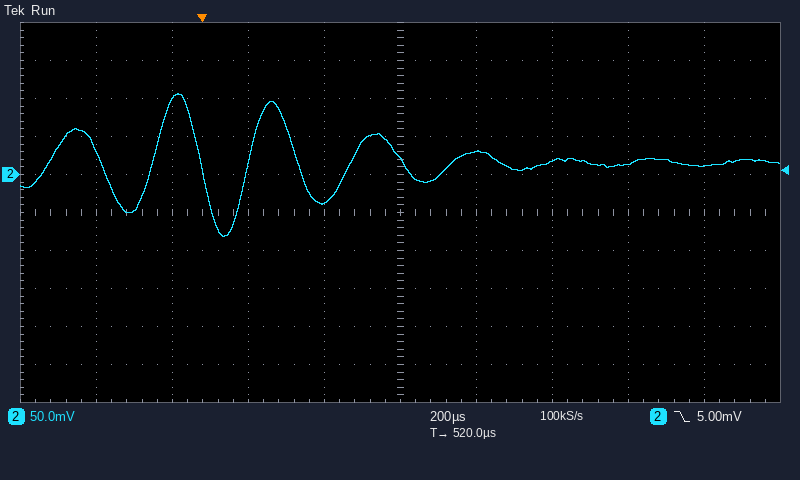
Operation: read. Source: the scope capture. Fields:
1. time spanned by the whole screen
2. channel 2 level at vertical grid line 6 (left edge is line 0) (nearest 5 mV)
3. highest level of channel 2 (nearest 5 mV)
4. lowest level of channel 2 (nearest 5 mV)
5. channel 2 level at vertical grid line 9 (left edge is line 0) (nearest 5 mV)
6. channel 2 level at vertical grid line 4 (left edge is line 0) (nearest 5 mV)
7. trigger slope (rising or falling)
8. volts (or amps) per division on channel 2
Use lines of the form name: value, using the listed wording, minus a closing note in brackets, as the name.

time spanned by the whole screen: 2 ms
channel 2 level at vertical grid line 6 (left edge is line 0): 30 mV
highest level of channel 2: 105 mV
lowest level of channel 2: -80 mV
channel 2 level at vertical grid line 9 (left edge is line 0): 10 mV
channel 2 level at vertical grid line 4 (left edge is line 0): -35 mV
trigger slope: falling
volts (or amps) per division on channel 2: 50 mV
